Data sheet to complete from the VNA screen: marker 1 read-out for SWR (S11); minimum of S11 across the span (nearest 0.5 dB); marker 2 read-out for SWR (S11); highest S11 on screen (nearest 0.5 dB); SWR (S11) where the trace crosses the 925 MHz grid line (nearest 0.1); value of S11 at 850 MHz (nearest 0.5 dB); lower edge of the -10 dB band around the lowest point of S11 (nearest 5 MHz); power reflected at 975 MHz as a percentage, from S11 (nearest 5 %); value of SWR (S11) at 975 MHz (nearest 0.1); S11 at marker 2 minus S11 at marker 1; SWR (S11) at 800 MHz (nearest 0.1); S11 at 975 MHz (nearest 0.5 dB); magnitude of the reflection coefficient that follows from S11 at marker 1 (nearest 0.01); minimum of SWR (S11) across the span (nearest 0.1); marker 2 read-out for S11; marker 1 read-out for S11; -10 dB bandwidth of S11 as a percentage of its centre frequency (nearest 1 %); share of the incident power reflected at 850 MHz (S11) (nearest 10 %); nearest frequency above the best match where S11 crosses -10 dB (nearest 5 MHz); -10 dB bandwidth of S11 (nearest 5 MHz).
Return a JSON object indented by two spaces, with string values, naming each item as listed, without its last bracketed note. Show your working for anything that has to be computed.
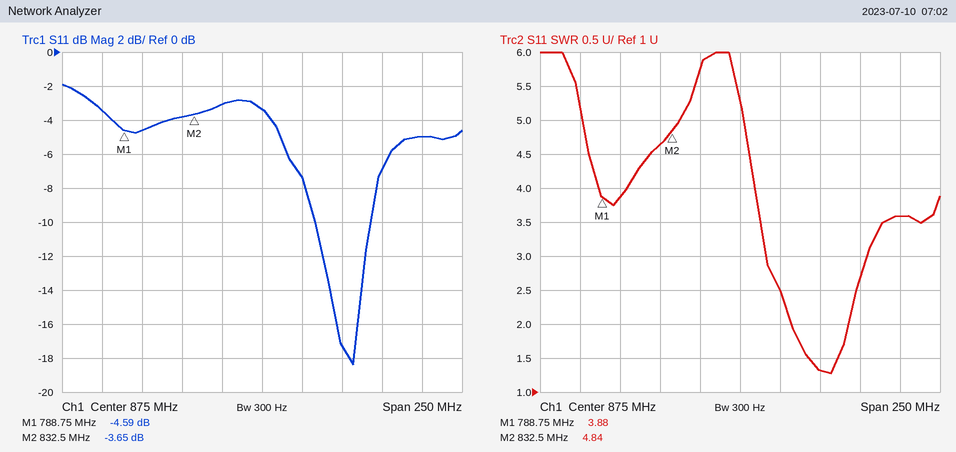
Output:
{
  "marker 1 read-out for SWR": "3.88",
  "minimum of S11 across the span": "-18.5 dB",
  "marker 2 read-out for SWR": "4.84",
  "highest S11 on screen": "-2.0 dB",
  "SWR (S11) where the trace crosses the 925 MHz grid line": "1.3",
  "value of S11 at 850 MHz": "-3.0 dB",
  "lower edge of the -10 dB band around the lowest point of S11": "910 MHz",
  "power reflected at 975 MHz as a percentage, from S11": "10^(-5/10) ≈ 31.6 %, so 30 % to the nearest 5 %",
  "value of SWR (S11) at 975 MHz": "3.6",
  "S11 at marker 2 minus S11 at marker 1": "-3.65 − (-4.59) = 0.94 dB",
  "SWR (S11) at 800 MHz": "3.9",
  "S11 at 975 MHz": "-5.0 dB",
  "magnitude of the reflection coefficient that follows from S11 at marker 1": "10^(-4.59/20) ≈ 0.59",
  "minimum of SWR (S11) across the span": "1.3",
  "marker 2 read-out for S11": "-3.65 dB",
  "marker 1 read-out for S11": "-4.59 dB",
  "-10 dB bandwidth of S11 as a percentage of its centre frequency": "35 MHz / 927.5 MHz ≈ 4 %",
  "share of the incident power reflected at 850 MHz (S11)": "10^(-3/10) ≈ 50 %",
  "nearest frequency above the best match where S11 crosses -10 dB": "945 MHz",
  "-10 dB bandwidth of S11": "945 MHz − 910 MHz = 35 MHz"
}
